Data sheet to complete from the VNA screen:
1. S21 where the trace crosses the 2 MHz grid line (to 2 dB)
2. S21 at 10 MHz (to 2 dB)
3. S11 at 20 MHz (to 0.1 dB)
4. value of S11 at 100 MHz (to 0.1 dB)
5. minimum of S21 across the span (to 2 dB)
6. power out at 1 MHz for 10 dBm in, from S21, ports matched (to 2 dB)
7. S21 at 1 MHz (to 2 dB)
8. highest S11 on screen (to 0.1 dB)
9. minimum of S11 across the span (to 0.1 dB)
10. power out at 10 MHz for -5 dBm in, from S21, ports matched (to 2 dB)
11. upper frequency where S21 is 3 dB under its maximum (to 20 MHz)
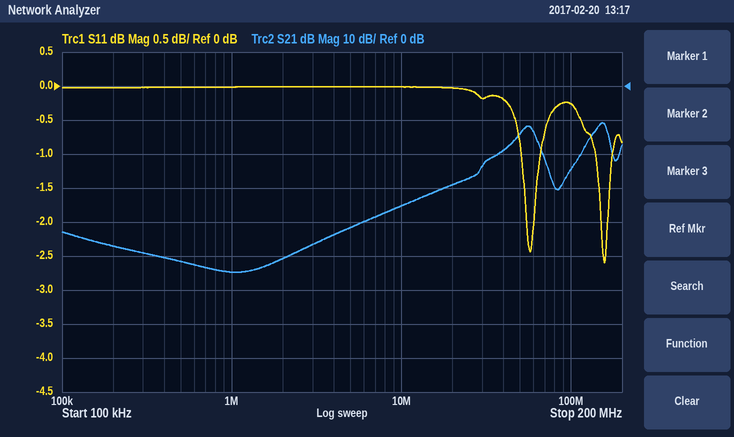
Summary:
-50 dB
-36 dB
0.0 dB
-0.3 dB
-54 dB
-44 dBm
-54 dB
0.0 dB
-2.6 dB
-40 dBm
160 MHz
